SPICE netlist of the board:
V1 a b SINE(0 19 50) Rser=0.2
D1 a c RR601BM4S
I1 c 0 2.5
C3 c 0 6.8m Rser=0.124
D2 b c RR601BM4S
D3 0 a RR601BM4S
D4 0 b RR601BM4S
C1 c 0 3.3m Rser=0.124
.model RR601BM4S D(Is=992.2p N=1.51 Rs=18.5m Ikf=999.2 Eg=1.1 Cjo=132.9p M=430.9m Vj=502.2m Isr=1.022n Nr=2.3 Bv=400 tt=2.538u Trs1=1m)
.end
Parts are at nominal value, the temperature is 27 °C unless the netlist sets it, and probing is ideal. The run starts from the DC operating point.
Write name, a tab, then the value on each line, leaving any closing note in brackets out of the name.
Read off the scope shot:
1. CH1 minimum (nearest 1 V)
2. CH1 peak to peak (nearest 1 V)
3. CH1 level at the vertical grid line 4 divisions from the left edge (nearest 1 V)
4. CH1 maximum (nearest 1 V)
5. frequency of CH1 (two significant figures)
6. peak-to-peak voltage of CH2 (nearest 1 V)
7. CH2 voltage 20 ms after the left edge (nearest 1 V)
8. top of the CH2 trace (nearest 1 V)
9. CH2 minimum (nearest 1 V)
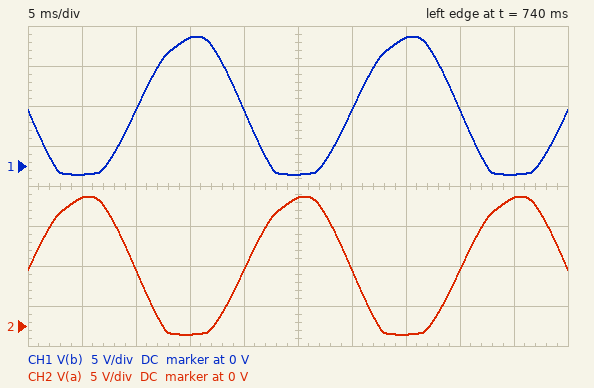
CH1 minimum	-1 V
CH1 peak to peak	17 V
CH1 level at the vertical grid line 4 divisions from the left edge	7 V
CH1 maximum	16 V
frequency of CH1	50 Hz
peak-to-peak voltage of CH2	17 V
CH2 voltage 20 ms after the left edge	7 V
top of the CH2 trace	16 V
CH2 minimum	-1 V
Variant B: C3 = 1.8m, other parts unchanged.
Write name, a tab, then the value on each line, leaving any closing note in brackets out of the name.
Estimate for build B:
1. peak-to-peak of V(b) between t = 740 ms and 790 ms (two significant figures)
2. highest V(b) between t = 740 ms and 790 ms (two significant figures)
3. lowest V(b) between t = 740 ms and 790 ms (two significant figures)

peak-to-peak of V(b) between t = 740 ms and 790 ms	18 V
highest V(b) between t = 740 ms and 790 ms	17 V
lowest V(b) between t = 740 ms and 790 ms	-1.1 V
